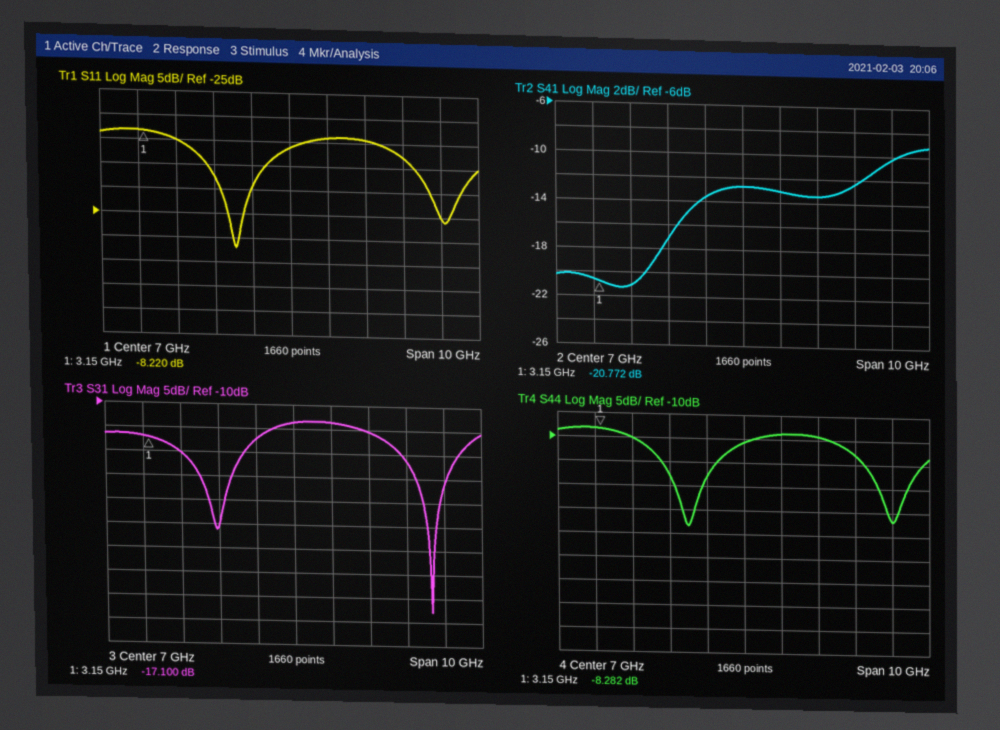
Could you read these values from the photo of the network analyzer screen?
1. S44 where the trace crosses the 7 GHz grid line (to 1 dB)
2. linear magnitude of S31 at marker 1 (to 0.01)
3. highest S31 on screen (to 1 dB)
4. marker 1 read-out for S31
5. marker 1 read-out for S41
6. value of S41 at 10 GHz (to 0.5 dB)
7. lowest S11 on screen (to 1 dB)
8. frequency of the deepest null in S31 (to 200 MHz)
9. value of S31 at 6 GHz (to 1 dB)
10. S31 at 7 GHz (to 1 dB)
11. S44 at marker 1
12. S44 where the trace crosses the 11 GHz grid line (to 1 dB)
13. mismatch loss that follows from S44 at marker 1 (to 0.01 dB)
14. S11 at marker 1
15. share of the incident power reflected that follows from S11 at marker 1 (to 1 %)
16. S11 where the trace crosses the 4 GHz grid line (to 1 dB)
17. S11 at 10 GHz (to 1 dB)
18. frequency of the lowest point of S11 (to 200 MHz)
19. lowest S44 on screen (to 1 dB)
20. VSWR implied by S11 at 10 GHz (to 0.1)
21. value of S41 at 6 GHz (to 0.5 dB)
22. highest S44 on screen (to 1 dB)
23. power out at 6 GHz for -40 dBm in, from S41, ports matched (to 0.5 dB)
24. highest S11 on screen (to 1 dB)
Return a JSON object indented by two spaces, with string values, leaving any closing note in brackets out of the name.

{
  "S44 where the trace crosses the 7 GHz grid line": "-11 dB",
  "linear magnitude of S31 at marker 1": "0.14",
  "highest S31 on screen": "-13 dB",
  "marker 1 read-out for S31": "-17.100 dB",
  "marker 1 read-out for S41": "-20.772 dB",
  "value of S41 at 10 GHz": "-12.5 dB",
  "lowest S11 on screen": "-32 dB",
  "frequency of the deepest null in S31": "10.6 GHz",
  "value of S31 at 6 GHz": "-17 dB",
  "S31 at 7 GHz": "-14 dB",
  "S44 at marker 1": "-8.282 dB",
  "S44 where the trace crosses the 11 GHz grid line": "-27 dB",
  "mismatch loss that follows from S44 at marker 1": "0.70 dB",
  "S11 at marker 1": "-8.220 dB",
  "share of the incident power reflected that follows from S11 at marker 1": "15 %",
  "S11 where the trace crosses the 4 GHz grid line": "-10 dB",
  "S11 at 10 GHz": "-13 dB",
  "frequency of the lowest point of S11": "5.6 GHz",
  "lowest S44 on screen": "-28 dB",
  "VSWR implied by S11 at 10 GHz": "1.6",
  "value of S41 at 6 GHz": "-13.5 dB",
  "highest S44 on screen": "-8 dB",
  "power out at 6 GHz for -40 dBm in, from S41, ports matched": "-53.5 dBm",
  "highest S11 on screen": "-8 dB"
}
